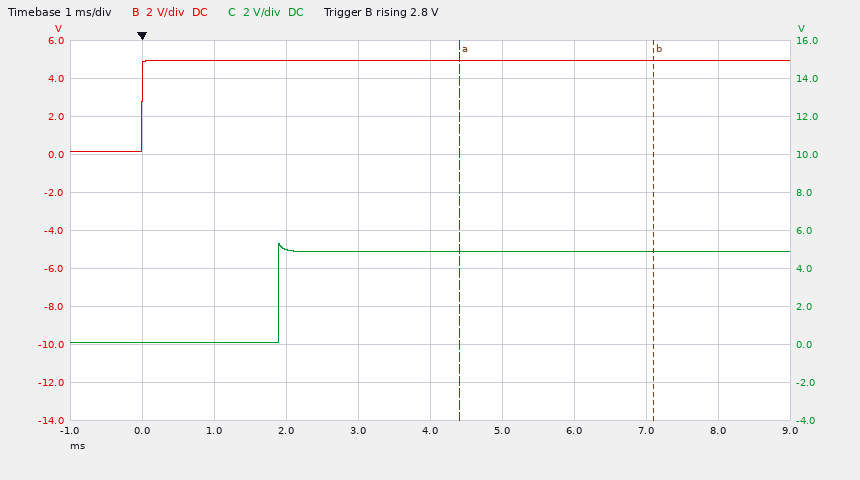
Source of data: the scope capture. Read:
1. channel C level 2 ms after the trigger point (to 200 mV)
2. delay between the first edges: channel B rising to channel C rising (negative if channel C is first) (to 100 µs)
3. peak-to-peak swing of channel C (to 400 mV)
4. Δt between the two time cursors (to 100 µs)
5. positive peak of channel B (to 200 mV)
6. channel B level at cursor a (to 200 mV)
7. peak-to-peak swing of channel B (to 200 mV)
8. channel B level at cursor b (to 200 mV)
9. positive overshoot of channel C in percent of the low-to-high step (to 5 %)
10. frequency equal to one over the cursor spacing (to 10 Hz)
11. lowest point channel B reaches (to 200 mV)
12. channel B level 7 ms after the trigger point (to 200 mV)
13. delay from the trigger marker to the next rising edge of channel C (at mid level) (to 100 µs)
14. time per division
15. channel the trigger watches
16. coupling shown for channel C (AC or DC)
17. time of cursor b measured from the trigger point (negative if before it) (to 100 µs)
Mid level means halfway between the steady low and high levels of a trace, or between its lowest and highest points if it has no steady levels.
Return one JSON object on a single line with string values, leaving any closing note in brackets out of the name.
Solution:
{"channel C level 2 ms after the trigger point": "5.0 V", "delay between the first edges: channel B rising to channel C rising (negative if channel C is first)": "+1.9 ms", "peak-to-peak swing of channel C": "5.2 V", "Δt between the two time cursors": "2.7 ms", "positive peak of channel B": "5.0 V", "channel B level at cursor a": "5.0 V", "peak-to-peak swing of channel B": "4.8 V", "channel B level at cursor b": "5.0 V", "positive overshoot of channel C in percent of the low-to-high step": "10 %", "frequency equal to one over the cursor spacing": "370 Hz", "lowest point channel B reaches": "200 mV", "channel B level 7 ms after the trigger point": "5.0 V", "delay from the trigger marker to the next rising edge of channel C (at mid level)": "1.9 ms", "time per division": "1 ms", "channel the trigger watches": "channel B", "coupling shown for channel C": "DC", "time of cursor b measured from the trigger point (negative if before it)": "+7.1 ms"}
